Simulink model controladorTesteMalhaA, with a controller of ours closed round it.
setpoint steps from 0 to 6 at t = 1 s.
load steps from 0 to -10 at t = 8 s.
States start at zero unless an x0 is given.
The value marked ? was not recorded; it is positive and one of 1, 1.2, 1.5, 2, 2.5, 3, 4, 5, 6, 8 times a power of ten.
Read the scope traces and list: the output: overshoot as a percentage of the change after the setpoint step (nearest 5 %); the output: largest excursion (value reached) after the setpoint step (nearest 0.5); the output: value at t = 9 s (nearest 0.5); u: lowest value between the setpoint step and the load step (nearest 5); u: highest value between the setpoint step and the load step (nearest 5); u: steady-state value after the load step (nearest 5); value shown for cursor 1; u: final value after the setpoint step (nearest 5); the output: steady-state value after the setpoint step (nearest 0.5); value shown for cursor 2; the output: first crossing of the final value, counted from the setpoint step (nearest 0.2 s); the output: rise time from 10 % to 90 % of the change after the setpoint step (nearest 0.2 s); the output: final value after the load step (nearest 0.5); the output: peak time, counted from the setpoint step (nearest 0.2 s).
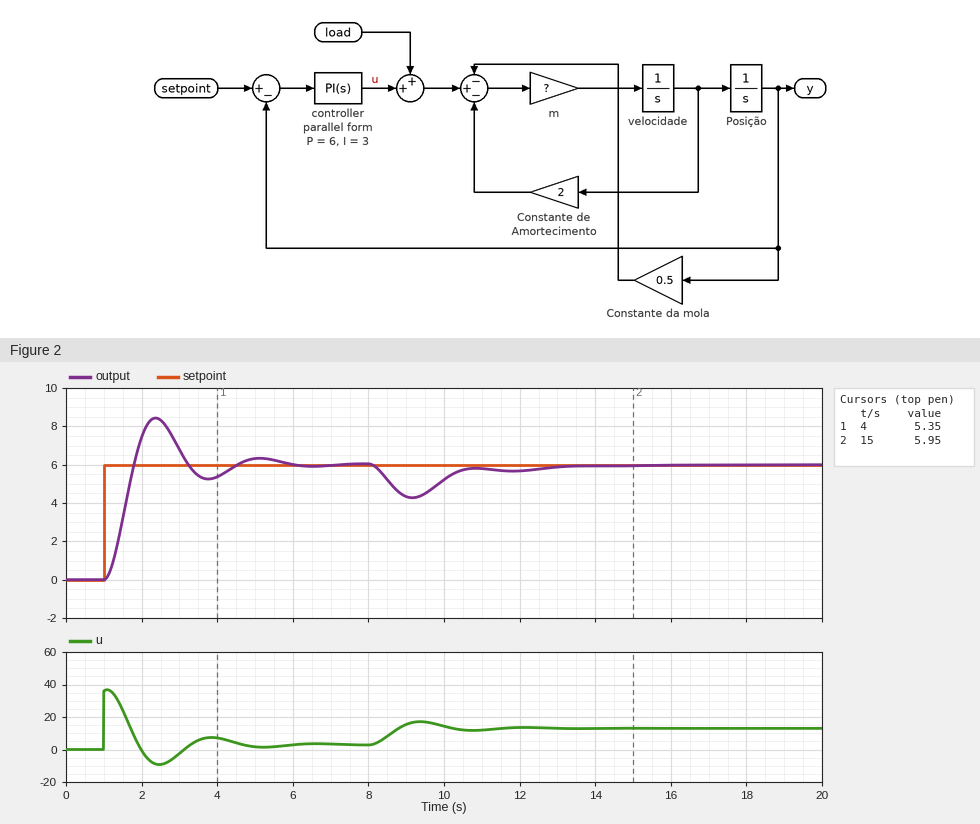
40 %
8.5
4.5
-10
35
15
5.35
5
6.0
5.95
0.8 s
0.6 s
6.0
1.4 s
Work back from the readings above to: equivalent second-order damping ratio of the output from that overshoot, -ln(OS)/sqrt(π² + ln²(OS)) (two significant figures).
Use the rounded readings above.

0.28
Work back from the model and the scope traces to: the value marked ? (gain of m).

1
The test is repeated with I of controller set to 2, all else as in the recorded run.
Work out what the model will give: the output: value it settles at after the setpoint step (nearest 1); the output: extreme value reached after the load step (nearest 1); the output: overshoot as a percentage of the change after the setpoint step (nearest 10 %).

6
4
30 %
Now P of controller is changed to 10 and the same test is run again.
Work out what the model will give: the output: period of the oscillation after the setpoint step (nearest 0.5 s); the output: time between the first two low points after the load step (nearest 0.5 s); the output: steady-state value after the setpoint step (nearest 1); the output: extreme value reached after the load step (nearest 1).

2.0 s
2.0 s
6
5
